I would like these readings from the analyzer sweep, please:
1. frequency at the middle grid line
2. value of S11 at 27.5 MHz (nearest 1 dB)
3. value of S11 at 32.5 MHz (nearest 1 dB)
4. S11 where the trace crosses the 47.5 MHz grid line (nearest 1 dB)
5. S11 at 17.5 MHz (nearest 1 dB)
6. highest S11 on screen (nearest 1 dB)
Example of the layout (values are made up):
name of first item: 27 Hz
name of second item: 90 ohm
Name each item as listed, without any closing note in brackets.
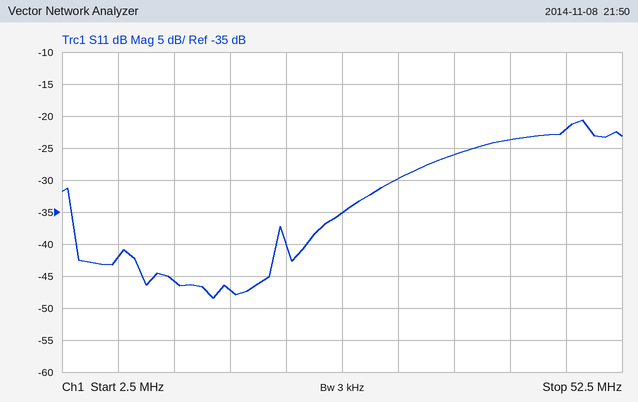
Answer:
frequency at the middle grid line: 27.5 MHz
value of S11 at 27.5 MHz: -35 dB
value of S11 at 32.5 MHz: -30 dB
S11 where the trace crosses the 47.5 MHz grid line: -22 dB
S11 at 17.5 MHz: -47 dB
highest S11 on screen: -21 dB
